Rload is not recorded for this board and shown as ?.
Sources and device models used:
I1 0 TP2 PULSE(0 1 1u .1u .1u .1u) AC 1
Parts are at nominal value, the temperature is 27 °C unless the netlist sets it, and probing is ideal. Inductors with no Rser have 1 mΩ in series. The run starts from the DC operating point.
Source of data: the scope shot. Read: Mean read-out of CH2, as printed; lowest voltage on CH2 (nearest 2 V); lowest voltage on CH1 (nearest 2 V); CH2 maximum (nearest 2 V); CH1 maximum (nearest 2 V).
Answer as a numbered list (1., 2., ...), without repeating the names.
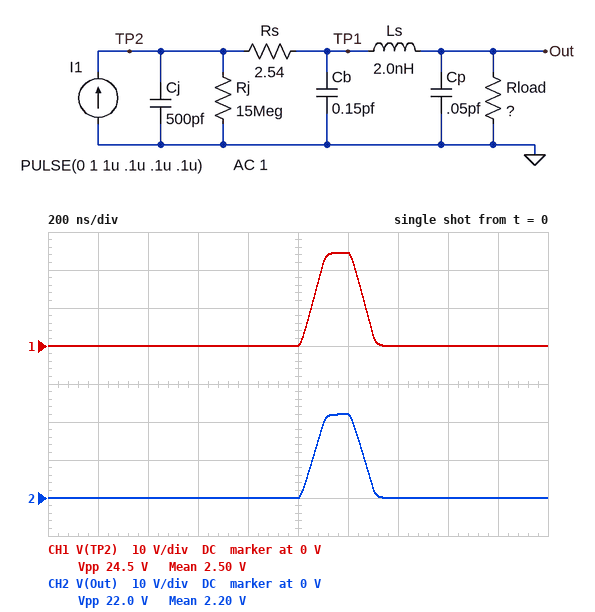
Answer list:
1. 2.20 V
2. 0 V
3. 0 V
4. 22 V
5. 24 V
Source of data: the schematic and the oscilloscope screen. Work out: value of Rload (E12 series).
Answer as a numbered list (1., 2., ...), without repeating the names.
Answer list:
1. 22 Ω
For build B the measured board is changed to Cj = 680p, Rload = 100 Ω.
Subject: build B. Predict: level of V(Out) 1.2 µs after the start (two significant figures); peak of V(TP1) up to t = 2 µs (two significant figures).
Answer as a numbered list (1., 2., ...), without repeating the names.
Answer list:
1. 87 V
2. 88 V
